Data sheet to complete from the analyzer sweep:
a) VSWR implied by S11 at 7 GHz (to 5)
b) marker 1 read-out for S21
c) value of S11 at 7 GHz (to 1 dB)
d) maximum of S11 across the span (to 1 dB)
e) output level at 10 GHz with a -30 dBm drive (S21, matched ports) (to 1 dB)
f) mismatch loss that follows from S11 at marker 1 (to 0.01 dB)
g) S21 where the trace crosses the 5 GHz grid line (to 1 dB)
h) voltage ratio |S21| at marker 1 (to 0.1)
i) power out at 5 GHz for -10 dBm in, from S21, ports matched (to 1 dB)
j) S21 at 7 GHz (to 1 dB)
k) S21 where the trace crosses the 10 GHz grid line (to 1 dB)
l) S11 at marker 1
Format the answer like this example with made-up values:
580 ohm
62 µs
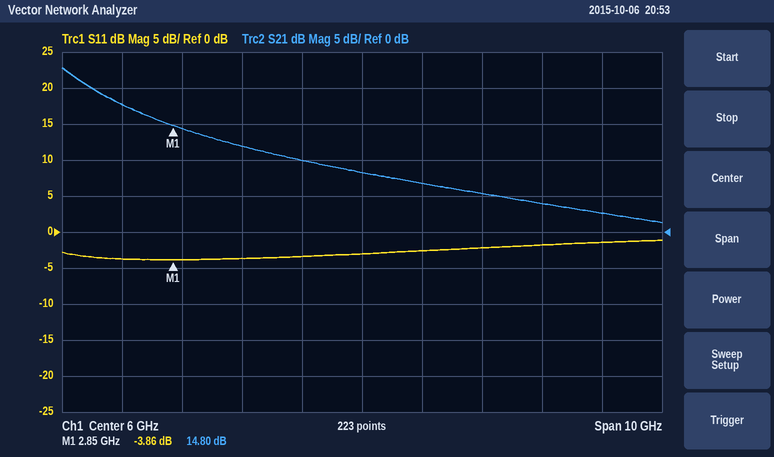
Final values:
5
14.80 dB
-3 dB
-1 dB
-27 dBm
2.30 dB
10 dB
5.5
0 dBm
7 dB
3 dB
-3.86 dB
